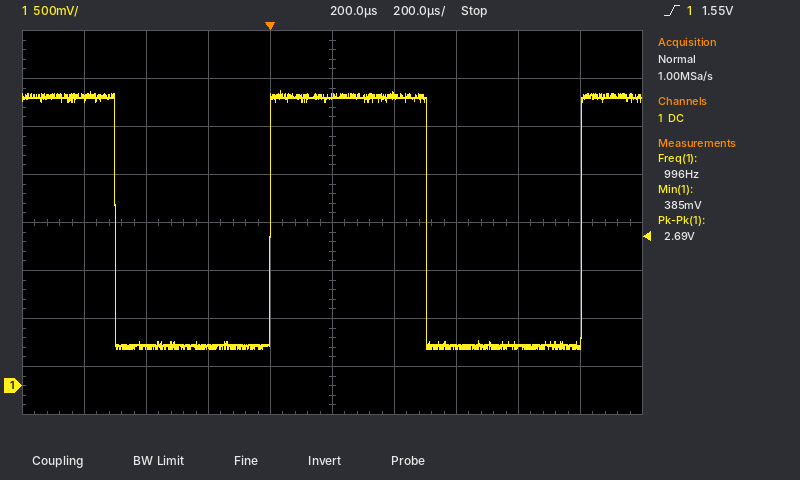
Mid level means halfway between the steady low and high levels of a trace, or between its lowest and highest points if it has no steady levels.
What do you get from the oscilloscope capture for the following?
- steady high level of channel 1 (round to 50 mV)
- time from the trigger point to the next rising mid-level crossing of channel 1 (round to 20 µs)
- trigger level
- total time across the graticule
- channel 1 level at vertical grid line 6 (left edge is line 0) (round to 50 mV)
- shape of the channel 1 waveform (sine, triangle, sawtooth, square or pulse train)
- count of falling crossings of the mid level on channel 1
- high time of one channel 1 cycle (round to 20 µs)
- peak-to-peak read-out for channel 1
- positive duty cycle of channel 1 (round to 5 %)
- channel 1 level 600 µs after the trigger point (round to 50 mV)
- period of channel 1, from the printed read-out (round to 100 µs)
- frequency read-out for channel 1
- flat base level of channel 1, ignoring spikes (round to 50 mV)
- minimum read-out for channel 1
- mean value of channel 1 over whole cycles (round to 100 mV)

3.00 V
1.00 ms
1.55 V
2 ms
3.05 V
square
2
500 µs
2.69 V
50 %
400 mV
1.0 ms
996 Hz
400 mV
385 mV
1.7 V
